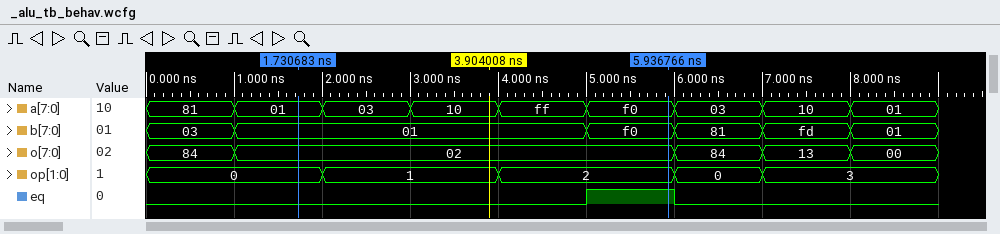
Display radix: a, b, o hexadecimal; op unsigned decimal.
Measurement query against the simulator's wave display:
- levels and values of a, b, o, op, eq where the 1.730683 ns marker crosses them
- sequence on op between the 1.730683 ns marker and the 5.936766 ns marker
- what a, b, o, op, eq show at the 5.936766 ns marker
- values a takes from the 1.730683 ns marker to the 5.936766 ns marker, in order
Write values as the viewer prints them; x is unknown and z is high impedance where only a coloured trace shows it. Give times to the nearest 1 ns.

a=01, b=01, o=02, op=0, eq=0
0, 1, 2
a=f0, b=f0, o=02, op=2, eq=1
01, 03, 10, ff, f0
